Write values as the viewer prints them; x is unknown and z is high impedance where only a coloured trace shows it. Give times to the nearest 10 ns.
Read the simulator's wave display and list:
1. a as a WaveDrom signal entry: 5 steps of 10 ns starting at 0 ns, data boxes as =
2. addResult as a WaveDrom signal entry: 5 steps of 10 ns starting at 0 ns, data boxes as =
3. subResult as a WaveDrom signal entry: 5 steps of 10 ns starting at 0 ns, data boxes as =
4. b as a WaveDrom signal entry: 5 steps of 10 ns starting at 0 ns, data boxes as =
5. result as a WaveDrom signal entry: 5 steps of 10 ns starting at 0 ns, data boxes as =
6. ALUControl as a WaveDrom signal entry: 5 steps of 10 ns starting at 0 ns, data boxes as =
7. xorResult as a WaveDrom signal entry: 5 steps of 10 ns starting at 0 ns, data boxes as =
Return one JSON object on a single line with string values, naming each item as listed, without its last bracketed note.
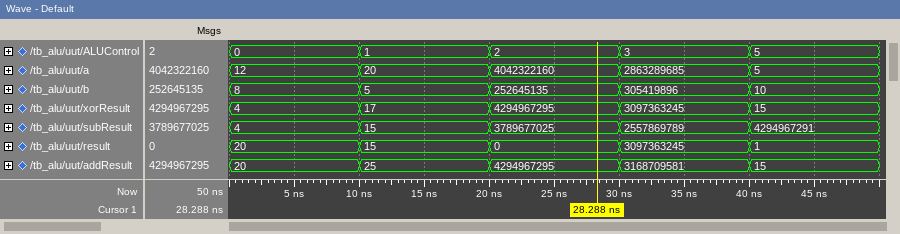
{"a as a WaveDrom signal entry: 5 steps of 10 ns starting at 0 ns, data boxes as =": "{name: 'a', wave: '=====', data: '12 20 4042322160 2863289685 5'}", "addResult as a WaveDrom signal entry: 5 steps of 10 ns starting at 0 ns, data boxes as =": "{name: 'addResult', wave: '=====', data: '20 25 4294967295 3168709581 15'}", "subResult as a WaveDrom signal entry: 5 steps of 10 ns starting at 0 ns, data boxes as =": "{name: 'subResult', wave: '=====', data: '4 15 3789677025 2557869789 4294967291'}", "b as a WaveDrom signal entry: 5 steps of 10 ns starting at 0 ns, data boxes as =": "{name: 'b', wave: '=====', data: '8 5 252645135 305419896 10'}", "result as a WaveDrom signal entry: 5 steps of 10 ns starting at 0 ns, data boxes as =": "{name: 'result', wave: '=====', data: '20 15 0 3097363245 1'}", "ALUControl as a WaveDrom signal entry: 5 steps of 10 ns starting at 0 ns, data boxes as =": "{name: 'ALUControl', wave: '=====', data: '0 1 2 3 5'}", "xorResult as a WaveDrom signal entry: 5 steps of 10 ns starting at 0 ns, data boxes as =": "{name: 'xorResult', wave: '=====', data: '4 17 4294967295 3097363245 15'}"}
